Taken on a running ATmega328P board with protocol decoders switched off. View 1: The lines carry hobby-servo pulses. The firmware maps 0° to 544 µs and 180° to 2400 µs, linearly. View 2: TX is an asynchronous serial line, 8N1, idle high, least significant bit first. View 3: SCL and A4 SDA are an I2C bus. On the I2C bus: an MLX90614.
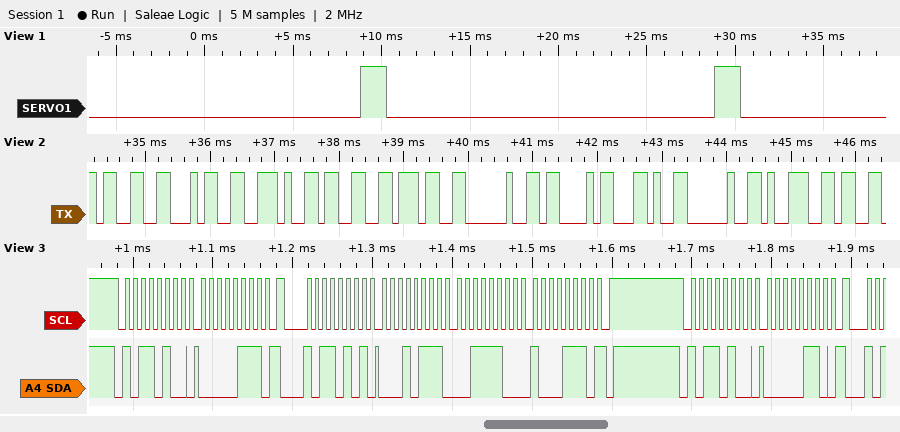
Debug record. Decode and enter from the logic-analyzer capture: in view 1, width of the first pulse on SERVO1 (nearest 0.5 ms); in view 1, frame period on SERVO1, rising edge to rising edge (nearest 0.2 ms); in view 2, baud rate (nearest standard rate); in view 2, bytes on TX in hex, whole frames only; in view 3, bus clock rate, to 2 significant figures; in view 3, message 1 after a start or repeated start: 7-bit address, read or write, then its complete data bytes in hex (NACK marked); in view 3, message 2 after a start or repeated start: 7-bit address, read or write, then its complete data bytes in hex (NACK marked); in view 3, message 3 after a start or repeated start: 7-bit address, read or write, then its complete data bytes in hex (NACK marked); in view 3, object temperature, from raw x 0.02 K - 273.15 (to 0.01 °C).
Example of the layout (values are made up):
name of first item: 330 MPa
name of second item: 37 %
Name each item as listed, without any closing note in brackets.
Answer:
in view 1, width of the first pulse on SERVO1: 1.5 ms
in view 1, frame period on SERVO1, rising edge to rising edge: 20.0 ms
in view 2, baud rate: 9600 baud
in view 2, bytes on TX in hex, whole frames only: 33 34 2E 33 37 20 43 2C 20 39
in view 3, bus clock rate, to 2 significant figures: 100 kHz
in view 3, message 1 after a start or repeated start: 7-bit address, read or write, then its complete data bytes in hex: 0x5A write: 07
in view 3, message 2 after a start or repeated start: 7-bit address, read or write, then its complete data bytes in hex: 0x5A read: 17 3C 8E NACK
in view 3, message 3 after a start or repeated start: 7-bit address, read or write, then its complete data bytes in hex: 0x5A write: 06
in view 3, object temperature, from raw x 0.02 K - 273.15: 34.51 °C
